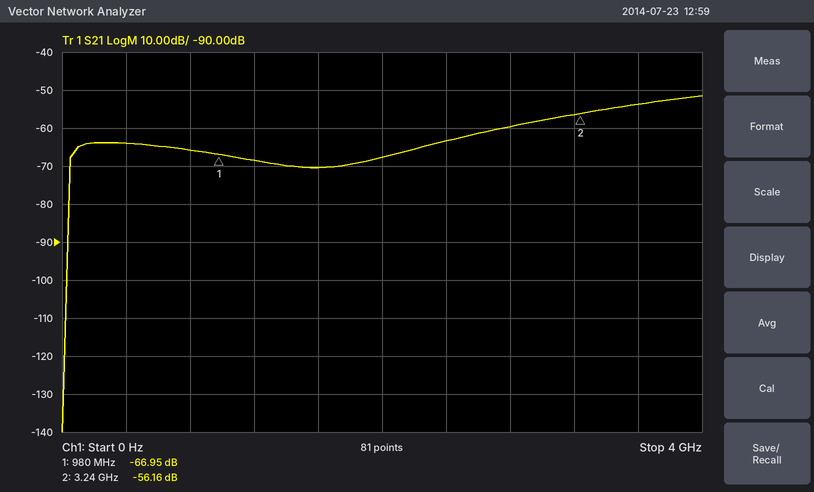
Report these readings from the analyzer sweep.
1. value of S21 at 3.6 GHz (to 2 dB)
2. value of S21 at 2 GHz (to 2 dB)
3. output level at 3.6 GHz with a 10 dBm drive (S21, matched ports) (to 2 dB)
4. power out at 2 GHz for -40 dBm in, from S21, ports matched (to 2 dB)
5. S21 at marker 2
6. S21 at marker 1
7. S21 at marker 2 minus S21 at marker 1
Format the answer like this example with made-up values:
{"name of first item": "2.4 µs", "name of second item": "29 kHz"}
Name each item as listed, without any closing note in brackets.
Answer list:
{"value of S21 at 3.6 GHz": "-54 dB", "value of S21 at 2 GHz": "-68 dB", "output level at 3.6 GHz with a 10 dBm drive (S21, matched ports)": "-44 dBm", "power out at 2 GHz for -40 dBm in, from S21, ports matched": "-108 dBm", "S21 at marker 2": "-56.16 dB", "S21 at marker 1": "-66.95 dB", "S21 at marker 2 minus S21 at marker 1": "10.79 dB"}
